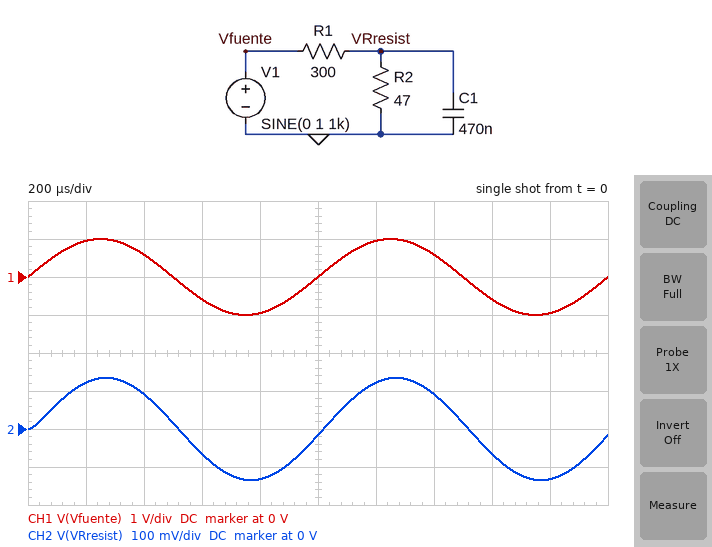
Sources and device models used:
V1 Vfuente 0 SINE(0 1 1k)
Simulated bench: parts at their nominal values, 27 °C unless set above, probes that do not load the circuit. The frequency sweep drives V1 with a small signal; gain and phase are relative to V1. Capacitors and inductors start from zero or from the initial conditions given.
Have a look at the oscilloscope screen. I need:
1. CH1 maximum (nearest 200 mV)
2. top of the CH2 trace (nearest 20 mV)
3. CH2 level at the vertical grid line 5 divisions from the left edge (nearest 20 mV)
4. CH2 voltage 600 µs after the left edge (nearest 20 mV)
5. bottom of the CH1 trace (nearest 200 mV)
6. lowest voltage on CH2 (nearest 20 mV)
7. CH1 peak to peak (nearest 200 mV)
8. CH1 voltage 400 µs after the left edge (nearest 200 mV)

1.0 V
140 mV
-20 mV
-60 mV
-1.0 V
-140 mV
2.0 V
600 mV
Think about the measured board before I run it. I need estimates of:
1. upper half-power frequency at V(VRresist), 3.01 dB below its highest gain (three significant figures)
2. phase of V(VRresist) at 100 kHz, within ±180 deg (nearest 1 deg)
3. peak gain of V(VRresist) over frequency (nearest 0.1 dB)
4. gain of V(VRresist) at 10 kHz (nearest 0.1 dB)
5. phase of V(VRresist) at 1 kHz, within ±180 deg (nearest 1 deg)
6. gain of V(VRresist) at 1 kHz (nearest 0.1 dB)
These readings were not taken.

8.33 kHz
-85 deg
-17.4 dB
-21.2 dB
-7 deg
-17.4 dB
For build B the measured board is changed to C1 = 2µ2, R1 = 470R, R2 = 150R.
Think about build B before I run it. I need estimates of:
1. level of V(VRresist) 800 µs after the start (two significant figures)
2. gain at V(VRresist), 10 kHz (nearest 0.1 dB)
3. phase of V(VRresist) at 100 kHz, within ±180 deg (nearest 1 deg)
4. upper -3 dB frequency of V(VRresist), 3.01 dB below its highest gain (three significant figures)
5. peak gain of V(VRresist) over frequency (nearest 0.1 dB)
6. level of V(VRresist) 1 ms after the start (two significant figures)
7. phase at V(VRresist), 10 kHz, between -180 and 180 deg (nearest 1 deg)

-96 mV
-36.3 dB
-90 deg
636 Hz
-12.3 dB
-110 mV
-86 deg
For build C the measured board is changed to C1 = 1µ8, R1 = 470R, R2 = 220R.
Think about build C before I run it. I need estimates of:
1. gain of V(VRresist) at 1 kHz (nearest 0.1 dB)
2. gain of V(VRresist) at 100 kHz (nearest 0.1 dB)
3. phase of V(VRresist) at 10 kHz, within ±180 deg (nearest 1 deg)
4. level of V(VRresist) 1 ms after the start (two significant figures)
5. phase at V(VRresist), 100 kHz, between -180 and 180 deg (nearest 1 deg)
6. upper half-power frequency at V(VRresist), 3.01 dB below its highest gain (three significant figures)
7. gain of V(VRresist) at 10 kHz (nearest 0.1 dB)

-15.8 dB
-54.5 dB
-87 deg
-140 mV
-90 deg
590 Hz
-34.5 dB
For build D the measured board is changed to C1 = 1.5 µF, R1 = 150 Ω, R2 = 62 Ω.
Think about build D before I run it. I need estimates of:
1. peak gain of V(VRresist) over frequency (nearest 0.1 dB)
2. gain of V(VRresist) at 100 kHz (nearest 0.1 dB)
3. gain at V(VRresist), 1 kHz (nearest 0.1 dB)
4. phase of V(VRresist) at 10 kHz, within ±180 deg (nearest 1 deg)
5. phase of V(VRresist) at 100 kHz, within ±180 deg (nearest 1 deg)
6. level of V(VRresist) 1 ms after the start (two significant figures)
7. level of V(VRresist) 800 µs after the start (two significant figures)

-10.7 dB
-43.0 dB
-11.4 dB
-76 deg
-89 deg
-100 mV
-270 mV
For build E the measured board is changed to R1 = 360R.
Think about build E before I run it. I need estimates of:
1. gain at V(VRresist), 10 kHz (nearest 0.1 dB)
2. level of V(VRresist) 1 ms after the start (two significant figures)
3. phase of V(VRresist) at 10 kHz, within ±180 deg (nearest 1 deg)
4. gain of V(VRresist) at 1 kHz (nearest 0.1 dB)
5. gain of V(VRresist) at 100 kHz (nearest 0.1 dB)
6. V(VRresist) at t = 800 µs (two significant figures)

-22.7 dB
-14 mV
-51 deg
-18.8 dB
-40.6 dB
-110 mV
